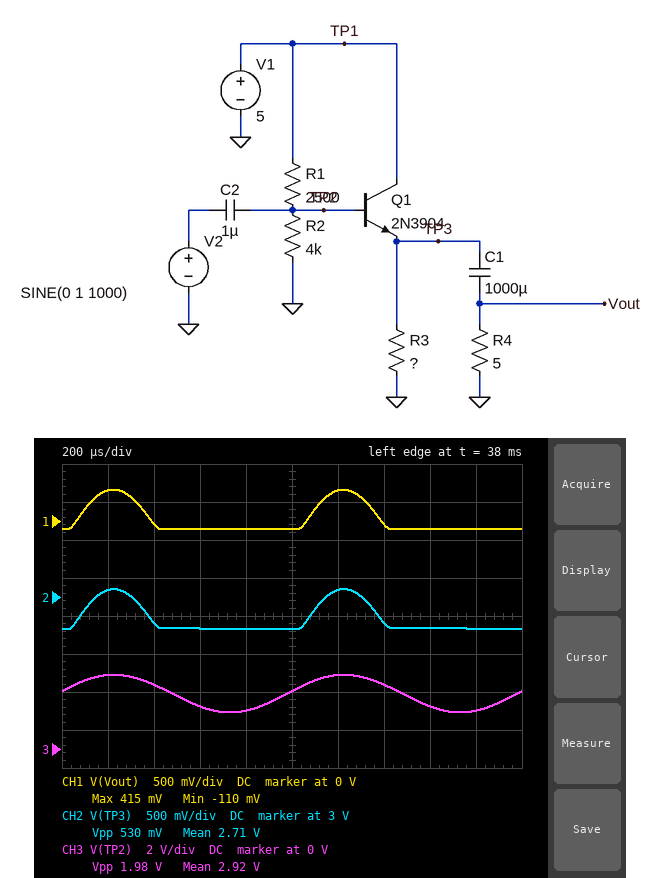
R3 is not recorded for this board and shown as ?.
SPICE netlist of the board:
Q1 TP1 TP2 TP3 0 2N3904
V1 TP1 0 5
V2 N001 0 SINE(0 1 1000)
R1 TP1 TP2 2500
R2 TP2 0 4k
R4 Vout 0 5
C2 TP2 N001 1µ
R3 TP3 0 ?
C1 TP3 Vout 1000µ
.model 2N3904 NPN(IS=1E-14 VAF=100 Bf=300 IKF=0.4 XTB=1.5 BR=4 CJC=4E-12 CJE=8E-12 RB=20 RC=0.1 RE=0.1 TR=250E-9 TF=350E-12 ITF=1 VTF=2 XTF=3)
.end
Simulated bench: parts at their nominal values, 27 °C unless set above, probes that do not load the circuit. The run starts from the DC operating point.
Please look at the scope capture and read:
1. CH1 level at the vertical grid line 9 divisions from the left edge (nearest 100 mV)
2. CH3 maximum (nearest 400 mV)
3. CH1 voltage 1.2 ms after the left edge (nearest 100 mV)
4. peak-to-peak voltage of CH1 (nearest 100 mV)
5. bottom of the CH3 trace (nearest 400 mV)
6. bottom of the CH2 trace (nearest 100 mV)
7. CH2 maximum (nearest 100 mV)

-100 mV
4.0 V
400 mV
500 mV
2.0 V
2.6 V
3.1 V
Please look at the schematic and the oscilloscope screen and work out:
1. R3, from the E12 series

120 Ω
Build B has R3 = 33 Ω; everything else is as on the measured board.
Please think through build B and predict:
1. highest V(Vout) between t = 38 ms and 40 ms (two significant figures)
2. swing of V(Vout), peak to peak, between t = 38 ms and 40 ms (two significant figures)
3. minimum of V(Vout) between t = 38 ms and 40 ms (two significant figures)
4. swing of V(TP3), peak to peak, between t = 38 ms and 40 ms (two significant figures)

610 mV
890 mV
-280 mV
900 mV
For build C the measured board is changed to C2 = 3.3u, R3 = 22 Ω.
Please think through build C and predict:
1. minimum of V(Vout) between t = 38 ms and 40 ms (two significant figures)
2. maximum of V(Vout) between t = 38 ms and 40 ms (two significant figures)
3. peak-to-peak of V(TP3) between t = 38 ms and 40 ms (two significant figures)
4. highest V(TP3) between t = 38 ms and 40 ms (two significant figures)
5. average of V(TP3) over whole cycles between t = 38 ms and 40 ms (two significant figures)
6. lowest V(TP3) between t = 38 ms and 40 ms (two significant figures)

-350 mV
670 mV
1.0 V
2.6 V
1.9 V
1.5 V
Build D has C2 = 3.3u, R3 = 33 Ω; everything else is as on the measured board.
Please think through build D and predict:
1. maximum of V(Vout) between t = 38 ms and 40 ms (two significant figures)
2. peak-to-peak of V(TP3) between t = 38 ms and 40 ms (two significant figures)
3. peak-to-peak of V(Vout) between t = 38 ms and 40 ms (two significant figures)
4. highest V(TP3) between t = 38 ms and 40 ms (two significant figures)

620 mV
910 mV
900 mV
2.8 V
